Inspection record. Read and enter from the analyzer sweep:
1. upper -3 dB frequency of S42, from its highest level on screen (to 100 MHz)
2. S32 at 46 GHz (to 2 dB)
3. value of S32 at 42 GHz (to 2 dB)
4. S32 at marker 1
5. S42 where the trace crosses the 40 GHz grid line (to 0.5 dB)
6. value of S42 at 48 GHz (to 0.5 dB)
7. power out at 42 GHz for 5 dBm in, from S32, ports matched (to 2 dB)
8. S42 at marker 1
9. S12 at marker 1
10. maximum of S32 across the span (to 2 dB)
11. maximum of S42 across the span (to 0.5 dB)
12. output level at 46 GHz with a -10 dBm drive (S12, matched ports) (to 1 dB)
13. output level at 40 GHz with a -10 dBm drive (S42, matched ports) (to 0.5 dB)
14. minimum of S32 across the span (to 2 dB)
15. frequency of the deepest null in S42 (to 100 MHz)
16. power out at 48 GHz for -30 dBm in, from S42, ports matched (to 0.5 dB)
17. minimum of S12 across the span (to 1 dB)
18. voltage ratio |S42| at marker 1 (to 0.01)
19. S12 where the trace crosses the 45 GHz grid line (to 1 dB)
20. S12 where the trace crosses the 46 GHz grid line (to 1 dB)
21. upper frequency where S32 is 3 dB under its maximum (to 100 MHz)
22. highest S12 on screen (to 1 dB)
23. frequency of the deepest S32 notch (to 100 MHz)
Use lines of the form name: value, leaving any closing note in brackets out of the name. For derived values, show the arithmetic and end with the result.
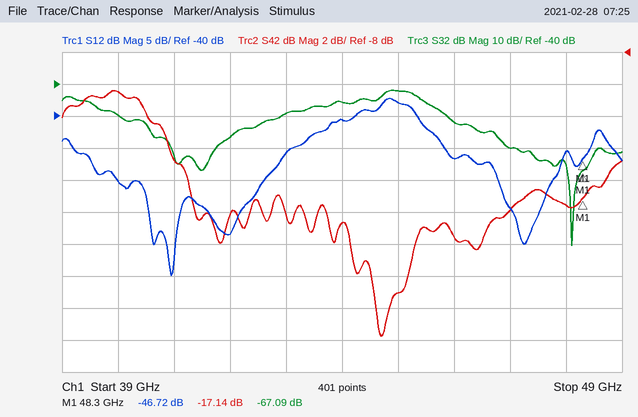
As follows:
upper -3 dB frequency of S42, from its highest level on screen: 40.9 GHz
S32 at 46 GHz: -52 dB
value of S32 at 42 GHz: -56 dB
S32 at marker 1: -67.09 dB
S42 where the trace crosses the 40 GHz grid line: -10.5 dB
value of S42 at 48 GHz: -17.5 dB
power out at 42 GHz for 5 dBm in, from S32, ports matched: 5 dBm + (-56 dB) = -52 dBm
S42 at marker 1: -17.14 dB
S12 at marker 1: -46.72 dB
maximum of S32 across the span: -42 dB
maximum of S42 across the span: -10.5 dB
output level at 46 GHz with a -10 dBm drive (S12, matched ports): -10 dBm + (-47 dB) = -57 dBm
output level at 40 GHz with a -10 dBm drive (S42, matched ports): -10 dBm + (-10.5 dB) = -20.5 dBm
minimum of S32 across the span: -90 dB
frequency of the deepest null in S42: 44.7 GHz
power out at 48 GHz for -30 dBm in, from S42, ports matched: -30 dBm + (-17.5 dB) = -47.5 dBm
minimum of S12 across the span: -65 dB
voltage ratio |S42| at marker 1: 10^(-17.14/20) ≈ 0.14
S12 where the trace crosses the 45 GHz grid line: -38 dB
S12 where the trace crosses the 46 GHz grid line: -47 dB
upper frequency where S32 is 3 dB under its maximum: 45.4 GHz
highest S12 on screen: -37 dB
frequency of the deepest S32 notch: 48.1 GHz
